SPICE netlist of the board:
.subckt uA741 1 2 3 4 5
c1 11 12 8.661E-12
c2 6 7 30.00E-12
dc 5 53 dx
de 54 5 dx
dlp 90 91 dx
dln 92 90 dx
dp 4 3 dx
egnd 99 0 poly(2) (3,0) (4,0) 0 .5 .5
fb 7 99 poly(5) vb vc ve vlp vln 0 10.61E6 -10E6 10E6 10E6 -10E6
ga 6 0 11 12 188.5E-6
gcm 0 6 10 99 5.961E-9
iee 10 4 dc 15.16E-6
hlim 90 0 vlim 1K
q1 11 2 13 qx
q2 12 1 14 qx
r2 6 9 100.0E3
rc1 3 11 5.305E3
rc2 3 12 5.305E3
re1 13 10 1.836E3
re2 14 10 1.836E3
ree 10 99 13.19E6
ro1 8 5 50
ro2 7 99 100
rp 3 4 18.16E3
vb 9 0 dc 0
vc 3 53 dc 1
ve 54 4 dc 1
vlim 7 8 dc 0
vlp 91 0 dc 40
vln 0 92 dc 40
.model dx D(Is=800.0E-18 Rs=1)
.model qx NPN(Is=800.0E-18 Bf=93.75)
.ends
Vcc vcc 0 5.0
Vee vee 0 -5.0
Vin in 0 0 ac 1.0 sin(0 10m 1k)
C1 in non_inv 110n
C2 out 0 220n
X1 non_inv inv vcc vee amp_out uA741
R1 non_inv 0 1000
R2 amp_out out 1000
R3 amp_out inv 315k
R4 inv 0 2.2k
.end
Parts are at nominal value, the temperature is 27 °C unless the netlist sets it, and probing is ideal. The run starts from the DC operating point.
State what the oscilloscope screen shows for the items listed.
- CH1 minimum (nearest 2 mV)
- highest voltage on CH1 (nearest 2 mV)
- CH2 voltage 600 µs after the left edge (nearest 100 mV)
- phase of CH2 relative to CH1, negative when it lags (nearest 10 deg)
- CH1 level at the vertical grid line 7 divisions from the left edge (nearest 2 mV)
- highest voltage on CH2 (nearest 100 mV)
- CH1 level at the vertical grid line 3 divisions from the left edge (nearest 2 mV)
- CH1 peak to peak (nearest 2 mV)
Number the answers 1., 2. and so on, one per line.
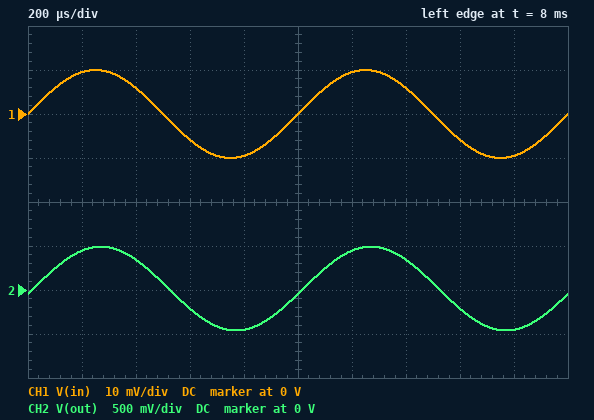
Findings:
1. -10 mV
2. 10 mV
3. -200 mV
4. -10 deg
5. 6 mV
6. 500 mV
7. -6 mV
8. 20 mV
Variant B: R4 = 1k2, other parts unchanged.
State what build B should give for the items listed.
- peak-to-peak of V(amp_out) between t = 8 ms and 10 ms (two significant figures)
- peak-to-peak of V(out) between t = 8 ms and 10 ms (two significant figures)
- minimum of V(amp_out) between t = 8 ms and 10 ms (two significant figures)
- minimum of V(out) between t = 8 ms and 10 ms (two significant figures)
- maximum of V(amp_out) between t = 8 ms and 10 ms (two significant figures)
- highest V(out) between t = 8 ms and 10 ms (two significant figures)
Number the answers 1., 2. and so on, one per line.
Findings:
1. 2.9 V
2. 1.7 V
3. -1.4 V
4. -840 mV
5. 1.5 V
6. 860 mV
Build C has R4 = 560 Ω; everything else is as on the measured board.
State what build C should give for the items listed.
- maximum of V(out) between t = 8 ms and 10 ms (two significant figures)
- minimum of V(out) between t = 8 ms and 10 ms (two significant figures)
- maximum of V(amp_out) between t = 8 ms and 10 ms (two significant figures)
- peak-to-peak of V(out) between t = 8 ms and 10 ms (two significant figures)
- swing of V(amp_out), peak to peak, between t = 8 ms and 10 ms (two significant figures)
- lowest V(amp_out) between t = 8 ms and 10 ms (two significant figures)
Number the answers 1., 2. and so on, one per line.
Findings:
1. 1.6 V
2. -1.6 V
3. 2.8 V
4. 3.3 V
5. 5.6 V
6. -2.8 V
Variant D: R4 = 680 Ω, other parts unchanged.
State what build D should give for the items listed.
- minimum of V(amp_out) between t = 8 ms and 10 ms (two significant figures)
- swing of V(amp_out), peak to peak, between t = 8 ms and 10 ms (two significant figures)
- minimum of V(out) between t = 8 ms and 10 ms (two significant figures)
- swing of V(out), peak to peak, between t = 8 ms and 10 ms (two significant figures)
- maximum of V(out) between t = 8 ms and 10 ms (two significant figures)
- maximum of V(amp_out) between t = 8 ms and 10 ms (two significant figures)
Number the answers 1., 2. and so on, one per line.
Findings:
1. -2.4 V
2. 4.8 V
3. -1.4 V
4. 2.8 V
5. 1.4 V
6. 2.4 V
